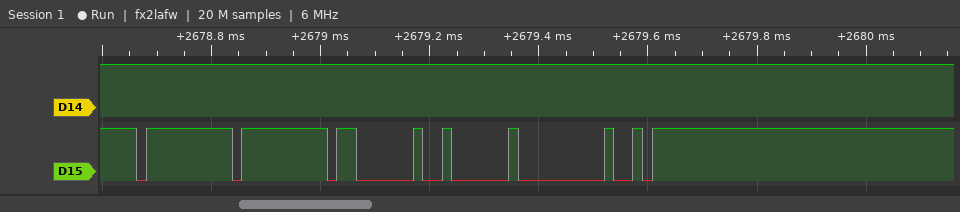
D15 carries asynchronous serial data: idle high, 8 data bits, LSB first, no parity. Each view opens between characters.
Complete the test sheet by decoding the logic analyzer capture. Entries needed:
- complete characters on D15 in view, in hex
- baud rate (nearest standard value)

FF, FF, 03, 02, 00, FA
57600 baud
